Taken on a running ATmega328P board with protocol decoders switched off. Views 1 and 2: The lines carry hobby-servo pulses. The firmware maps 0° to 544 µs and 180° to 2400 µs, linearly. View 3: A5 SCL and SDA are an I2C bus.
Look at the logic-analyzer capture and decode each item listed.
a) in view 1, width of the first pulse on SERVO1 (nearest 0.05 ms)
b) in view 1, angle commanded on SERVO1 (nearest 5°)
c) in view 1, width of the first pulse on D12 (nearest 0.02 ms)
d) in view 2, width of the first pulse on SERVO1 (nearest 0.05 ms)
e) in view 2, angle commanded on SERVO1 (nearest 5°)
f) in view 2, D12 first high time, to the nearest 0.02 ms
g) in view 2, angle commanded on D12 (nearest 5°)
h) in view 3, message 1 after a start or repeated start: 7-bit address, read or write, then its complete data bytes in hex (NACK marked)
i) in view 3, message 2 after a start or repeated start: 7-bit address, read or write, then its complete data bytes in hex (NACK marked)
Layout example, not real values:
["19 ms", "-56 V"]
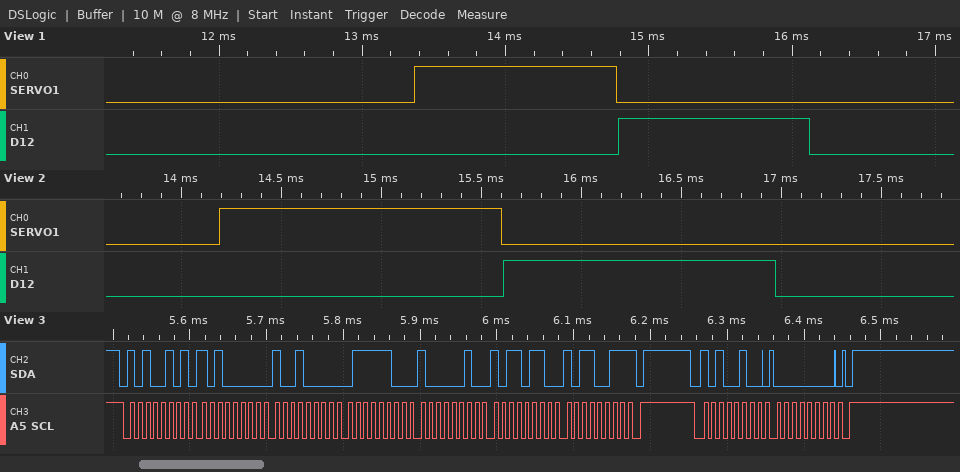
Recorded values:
["1.40 ms", "85°", "1.34 ms", "1.40 ms", "85°", "1.36 ms", "80°", "0x52 read: A0 90 7C 82 B6 B3 NACK", "0x52 write: 00"]
